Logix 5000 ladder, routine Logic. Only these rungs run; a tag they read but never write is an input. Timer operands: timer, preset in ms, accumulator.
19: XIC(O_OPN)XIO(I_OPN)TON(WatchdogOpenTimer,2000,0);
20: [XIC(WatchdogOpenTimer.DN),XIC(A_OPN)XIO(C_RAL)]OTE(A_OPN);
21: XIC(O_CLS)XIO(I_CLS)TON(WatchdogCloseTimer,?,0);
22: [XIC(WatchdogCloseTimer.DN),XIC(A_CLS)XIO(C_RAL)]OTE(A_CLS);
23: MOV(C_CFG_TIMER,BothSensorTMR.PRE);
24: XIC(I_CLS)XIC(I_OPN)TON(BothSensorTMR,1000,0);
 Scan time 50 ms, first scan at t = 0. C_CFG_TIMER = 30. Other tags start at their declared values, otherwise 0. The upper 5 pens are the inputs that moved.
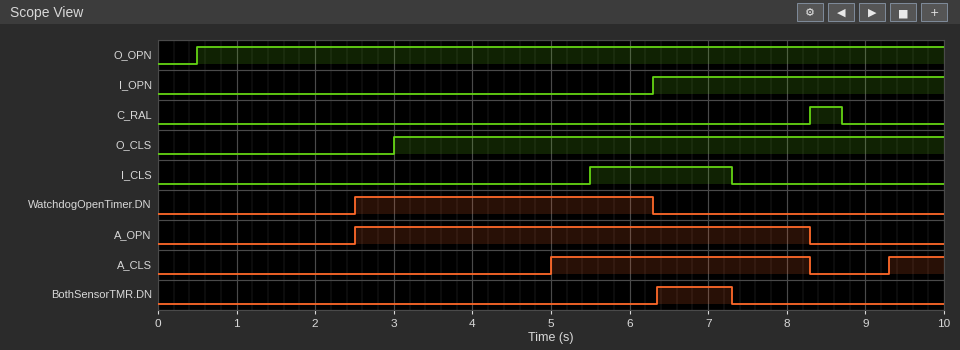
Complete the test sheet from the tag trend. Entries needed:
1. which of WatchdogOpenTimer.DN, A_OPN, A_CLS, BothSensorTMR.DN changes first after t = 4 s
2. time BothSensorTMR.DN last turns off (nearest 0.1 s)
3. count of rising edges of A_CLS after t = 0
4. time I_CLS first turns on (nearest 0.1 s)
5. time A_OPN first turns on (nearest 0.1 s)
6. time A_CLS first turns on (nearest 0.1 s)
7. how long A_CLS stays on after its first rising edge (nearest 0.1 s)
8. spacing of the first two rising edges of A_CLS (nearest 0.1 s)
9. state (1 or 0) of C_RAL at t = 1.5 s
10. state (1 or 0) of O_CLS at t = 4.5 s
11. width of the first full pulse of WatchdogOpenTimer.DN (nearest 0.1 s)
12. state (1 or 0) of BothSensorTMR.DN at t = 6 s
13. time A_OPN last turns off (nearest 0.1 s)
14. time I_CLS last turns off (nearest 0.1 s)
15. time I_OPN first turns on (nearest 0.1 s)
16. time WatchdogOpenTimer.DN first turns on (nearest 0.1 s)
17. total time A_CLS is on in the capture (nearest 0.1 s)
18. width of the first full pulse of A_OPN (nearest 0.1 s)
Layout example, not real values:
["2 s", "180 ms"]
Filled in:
["A_CLS", "7.3 s", "2", "5.5 s", "2.5 s", "5.0 s", "3.3 s", "4.3 s", "0", "1", "3.8 s", "0", "8.3 s", "7.3 s", "6.3 s", "2.5 s", "4.0 s", "5.8 s"]
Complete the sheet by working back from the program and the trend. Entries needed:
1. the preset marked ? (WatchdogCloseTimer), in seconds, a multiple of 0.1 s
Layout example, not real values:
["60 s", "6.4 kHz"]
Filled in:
["2.0 s"]
